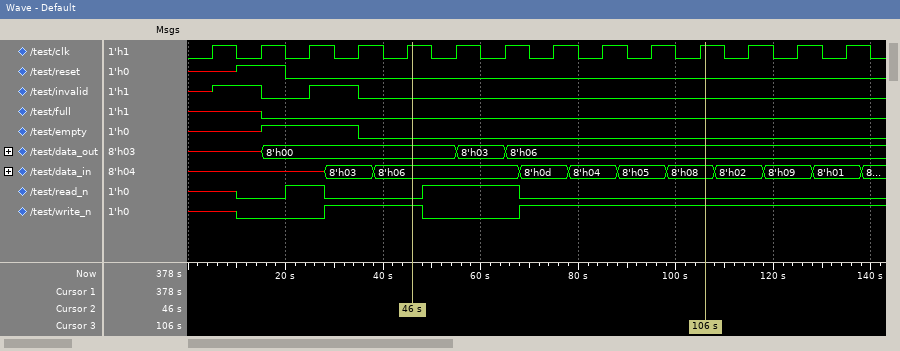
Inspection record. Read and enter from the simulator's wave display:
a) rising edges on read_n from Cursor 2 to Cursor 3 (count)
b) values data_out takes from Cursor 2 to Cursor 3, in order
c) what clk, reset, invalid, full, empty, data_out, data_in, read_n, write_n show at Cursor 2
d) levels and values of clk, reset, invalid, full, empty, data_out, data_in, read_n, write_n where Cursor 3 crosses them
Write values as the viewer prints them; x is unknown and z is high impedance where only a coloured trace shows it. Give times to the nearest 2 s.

1
8'h00, 8'h03, 8'h06
clk=1, reset=0, invalid=0, full=0, empty=0, data_out=8'h00, data_in=8'h06, read_n=0, write_n=1
clk=1, reset=0, invalid=0, full=0, empty=0, data_out=8'h06, data_in=8'h08, read_n=0, write_n=1
